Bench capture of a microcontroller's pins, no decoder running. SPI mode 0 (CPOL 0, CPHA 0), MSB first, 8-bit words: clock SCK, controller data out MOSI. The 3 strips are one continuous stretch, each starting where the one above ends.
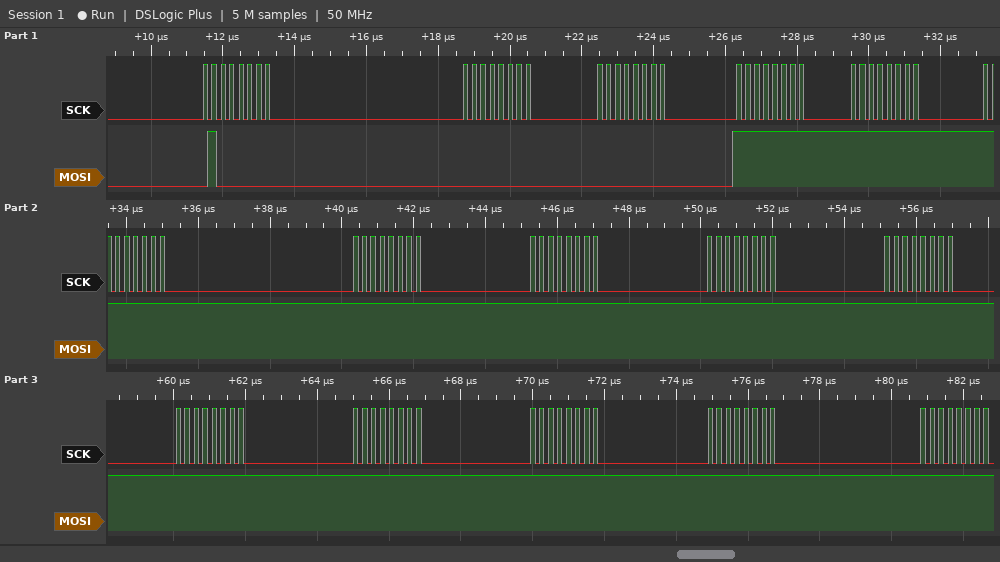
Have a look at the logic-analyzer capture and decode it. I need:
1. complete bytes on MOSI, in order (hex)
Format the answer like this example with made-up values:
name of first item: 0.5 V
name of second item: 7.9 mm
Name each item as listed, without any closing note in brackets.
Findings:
complete bytes on MOSI, in order: 40 00 00 FF FF FF FF FF FF FF FF FF FF FF FF
